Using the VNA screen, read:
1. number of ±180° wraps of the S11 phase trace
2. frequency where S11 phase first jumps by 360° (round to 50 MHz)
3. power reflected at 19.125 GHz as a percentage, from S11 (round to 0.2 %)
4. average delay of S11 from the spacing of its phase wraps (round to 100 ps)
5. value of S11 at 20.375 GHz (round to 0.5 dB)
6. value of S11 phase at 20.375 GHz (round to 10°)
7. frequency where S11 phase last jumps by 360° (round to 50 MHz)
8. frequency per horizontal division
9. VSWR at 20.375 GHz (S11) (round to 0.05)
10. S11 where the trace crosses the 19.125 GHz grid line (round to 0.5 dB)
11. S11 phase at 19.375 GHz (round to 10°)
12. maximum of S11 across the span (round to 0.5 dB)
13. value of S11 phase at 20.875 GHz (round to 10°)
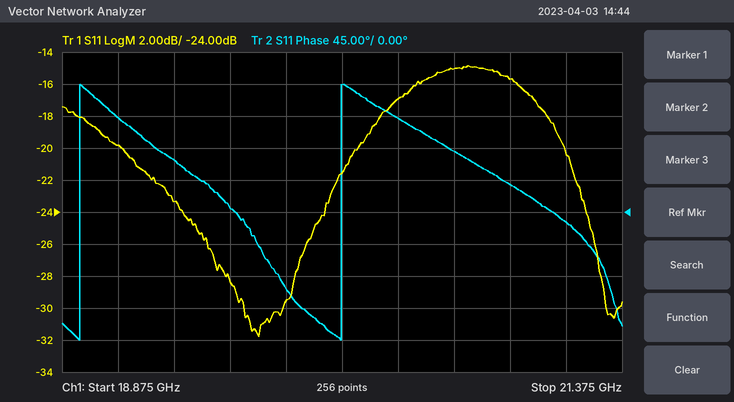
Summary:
2
18.95 GHz
1.0 %
900 ps
-17.0 dB
130°
20.10 GHz
250 MHz
1.35
-20.0 dB
70°
-15.0 dB
40°
